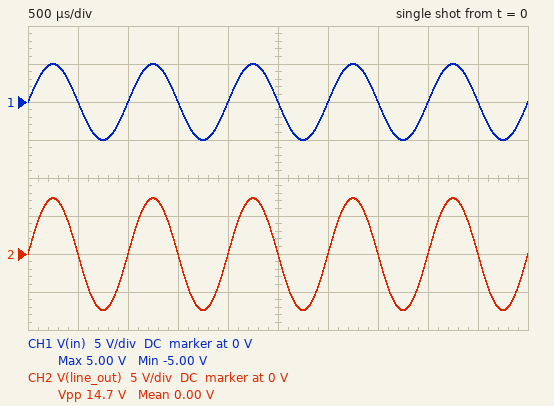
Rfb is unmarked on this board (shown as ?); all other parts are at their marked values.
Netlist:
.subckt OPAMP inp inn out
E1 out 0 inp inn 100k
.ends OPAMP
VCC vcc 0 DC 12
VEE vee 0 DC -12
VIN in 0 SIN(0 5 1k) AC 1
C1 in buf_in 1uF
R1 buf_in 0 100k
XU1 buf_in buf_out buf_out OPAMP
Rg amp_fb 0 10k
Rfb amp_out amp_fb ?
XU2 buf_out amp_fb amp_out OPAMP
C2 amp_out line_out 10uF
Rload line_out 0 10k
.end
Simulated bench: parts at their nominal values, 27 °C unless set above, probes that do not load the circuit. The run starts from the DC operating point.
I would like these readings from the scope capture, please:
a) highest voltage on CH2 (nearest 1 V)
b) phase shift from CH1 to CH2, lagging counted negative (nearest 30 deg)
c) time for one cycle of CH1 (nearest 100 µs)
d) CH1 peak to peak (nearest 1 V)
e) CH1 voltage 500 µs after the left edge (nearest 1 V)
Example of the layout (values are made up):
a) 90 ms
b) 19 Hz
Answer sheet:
a) 7 V
b) 0 deg
c) 1.0 ms
d) 10 V
e) 0 V
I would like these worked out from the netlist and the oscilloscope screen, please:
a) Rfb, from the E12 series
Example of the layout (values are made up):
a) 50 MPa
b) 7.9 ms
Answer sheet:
a) 4.7 kΩ
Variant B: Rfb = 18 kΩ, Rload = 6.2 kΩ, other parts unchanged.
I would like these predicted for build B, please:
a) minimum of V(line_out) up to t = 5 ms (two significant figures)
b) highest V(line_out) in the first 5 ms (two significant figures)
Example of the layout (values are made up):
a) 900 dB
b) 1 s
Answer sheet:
a) -14 V
b) 14 V
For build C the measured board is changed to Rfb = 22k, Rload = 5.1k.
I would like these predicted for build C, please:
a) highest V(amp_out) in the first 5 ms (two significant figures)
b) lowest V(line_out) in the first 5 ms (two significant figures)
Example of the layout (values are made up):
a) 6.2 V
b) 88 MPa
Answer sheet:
a) 16 V
b) -16 V
